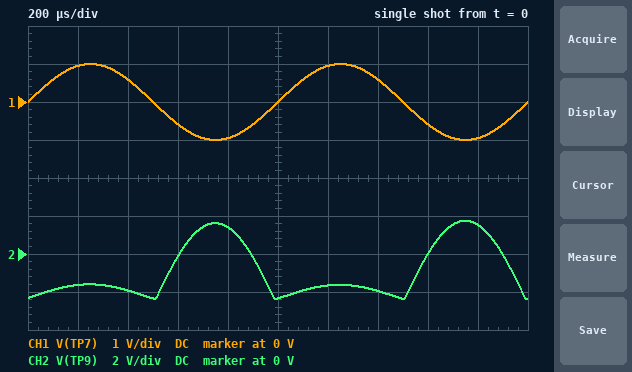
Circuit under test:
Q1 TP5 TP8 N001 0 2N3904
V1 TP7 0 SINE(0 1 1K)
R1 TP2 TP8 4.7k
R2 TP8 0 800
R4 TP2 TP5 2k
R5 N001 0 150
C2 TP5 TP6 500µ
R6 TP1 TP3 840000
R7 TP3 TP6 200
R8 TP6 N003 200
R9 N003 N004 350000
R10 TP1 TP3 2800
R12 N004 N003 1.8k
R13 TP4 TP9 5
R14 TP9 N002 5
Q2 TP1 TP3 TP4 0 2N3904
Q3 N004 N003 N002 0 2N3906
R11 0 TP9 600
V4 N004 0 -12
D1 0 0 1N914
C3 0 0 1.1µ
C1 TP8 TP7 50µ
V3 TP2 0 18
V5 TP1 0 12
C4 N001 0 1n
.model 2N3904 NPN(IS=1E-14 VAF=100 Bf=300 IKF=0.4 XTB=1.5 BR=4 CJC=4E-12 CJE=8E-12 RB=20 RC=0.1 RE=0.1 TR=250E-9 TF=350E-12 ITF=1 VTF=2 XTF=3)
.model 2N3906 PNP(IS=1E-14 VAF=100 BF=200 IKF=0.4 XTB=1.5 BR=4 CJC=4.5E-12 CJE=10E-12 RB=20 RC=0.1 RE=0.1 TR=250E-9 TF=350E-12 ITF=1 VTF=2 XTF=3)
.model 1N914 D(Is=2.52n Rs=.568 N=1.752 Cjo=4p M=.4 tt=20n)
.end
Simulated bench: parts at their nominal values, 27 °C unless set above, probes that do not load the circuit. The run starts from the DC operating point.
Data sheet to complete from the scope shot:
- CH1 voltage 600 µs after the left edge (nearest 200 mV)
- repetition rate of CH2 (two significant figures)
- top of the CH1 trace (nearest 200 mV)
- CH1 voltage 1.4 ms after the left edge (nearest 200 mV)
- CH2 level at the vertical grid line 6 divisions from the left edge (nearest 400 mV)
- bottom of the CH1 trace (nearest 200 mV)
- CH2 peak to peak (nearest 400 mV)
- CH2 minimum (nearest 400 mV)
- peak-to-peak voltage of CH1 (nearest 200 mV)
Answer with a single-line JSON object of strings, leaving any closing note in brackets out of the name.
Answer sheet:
{"CH1 voltage 600 µs after the left edge": "-600 mV", "repetition rate of CH2": "1.0 kHz", "top of the CH1 trace": "1.0 V", "CH1 voltage 1.4 ms after the left edge": "600 mV", "CH2 level at the vertical grid line 6 divisions from the left edge": "-1.6 V", "bottom of the CH1 trace": "-1.0 V", "CH2 peak to peak": "4.0 V", "CH2 minimum": "-2.4 V", "peak-to-peak voltage of CH1": "2.0 V"}
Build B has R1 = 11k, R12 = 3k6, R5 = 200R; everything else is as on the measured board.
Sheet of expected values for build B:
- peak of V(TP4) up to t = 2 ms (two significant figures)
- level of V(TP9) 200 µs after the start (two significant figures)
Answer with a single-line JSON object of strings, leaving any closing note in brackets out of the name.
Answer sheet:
{"peak of V(TP4) up to t = 2 ms": "3.6 V", "level of V(TP9) 200 µs after the start": "-2.5 V"}
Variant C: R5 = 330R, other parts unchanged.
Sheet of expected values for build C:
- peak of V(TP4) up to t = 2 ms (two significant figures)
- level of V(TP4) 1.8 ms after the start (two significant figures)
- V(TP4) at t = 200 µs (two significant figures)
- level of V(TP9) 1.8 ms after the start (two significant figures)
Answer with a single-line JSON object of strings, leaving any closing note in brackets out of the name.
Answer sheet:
{"peak of V(TP4) up to t = 2 ms": "-82 mV", "level of V(TP4) 1.8 ms after the start": "-190 mV", "V(TP4) at t = 200 µs": "-4.1 V", "level of V(TP9) 1.8 ms after the start": "-390 mV"}
